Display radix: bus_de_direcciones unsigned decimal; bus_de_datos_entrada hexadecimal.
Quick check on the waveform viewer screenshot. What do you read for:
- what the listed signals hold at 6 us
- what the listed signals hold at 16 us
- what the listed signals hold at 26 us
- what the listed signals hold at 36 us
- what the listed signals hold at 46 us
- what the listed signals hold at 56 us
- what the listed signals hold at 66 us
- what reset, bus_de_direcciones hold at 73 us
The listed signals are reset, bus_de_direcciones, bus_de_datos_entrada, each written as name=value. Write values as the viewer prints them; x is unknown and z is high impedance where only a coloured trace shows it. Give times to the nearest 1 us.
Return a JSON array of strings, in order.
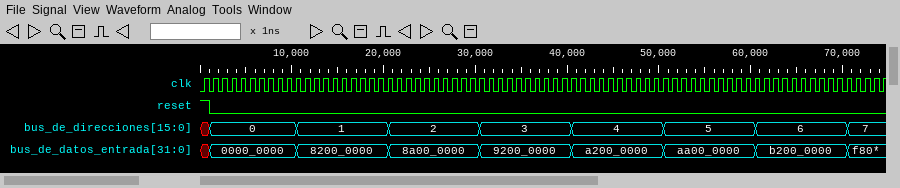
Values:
["reset=0, bus_de_direcciones=0, bus_de_datos_entrada=0000_0000", "reset=0, bus_de_direcciones=1, bus_de_datos_entrada=8200_0000", "reset=0, bus_de_direcciones=2, bus_de_datos_entrada=8a00_0000", "reset=0, bus_de_direcciones=3, bus_de_datos_entrada=9200_0000", "reset=0, bus_de_direcciones=4, bus_de_datos_entrada=a200_0000", "reset=0, bus_de_direcciones=5, bus_de_datos_entrada=aa00_0000", "reset=0, bus_de_direcciones=6, bus_de_datos_entrada=b200_0000", "reset=0, bus_de_direcciones=7"]
